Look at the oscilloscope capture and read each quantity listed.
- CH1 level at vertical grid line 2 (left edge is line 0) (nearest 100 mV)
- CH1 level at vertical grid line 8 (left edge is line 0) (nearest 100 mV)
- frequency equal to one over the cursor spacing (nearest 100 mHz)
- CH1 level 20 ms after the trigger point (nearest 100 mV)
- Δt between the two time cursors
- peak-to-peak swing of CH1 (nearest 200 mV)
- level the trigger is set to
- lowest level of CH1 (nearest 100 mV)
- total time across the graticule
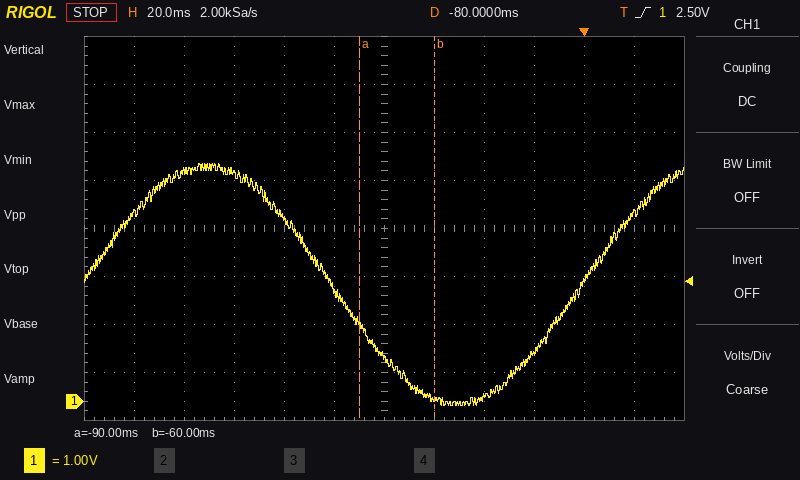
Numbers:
4.8 V
100 mV
33.3 Hz
3.9 V
30 ms
5.0 V
2.50 V
-100 mV
240 ms
